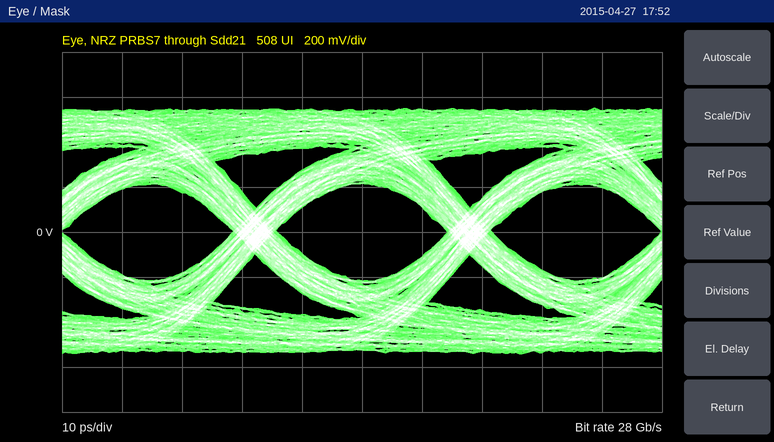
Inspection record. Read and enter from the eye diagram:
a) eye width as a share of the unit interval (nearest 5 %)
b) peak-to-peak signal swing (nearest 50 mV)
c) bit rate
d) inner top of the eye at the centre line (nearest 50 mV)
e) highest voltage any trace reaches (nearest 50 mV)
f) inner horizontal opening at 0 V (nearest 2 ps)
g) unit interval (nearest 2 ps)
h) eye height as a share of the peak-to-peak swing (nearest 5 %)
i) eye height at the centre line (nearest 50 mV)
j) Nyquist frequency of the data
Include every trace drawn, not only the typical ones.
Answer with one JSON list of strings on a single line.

["80 %", "1.10 V", "28 Gb/s", "200 mV", "550 mV", "28 ps", "36 ps", "40 %", "450 mV", "14 GHz"]
